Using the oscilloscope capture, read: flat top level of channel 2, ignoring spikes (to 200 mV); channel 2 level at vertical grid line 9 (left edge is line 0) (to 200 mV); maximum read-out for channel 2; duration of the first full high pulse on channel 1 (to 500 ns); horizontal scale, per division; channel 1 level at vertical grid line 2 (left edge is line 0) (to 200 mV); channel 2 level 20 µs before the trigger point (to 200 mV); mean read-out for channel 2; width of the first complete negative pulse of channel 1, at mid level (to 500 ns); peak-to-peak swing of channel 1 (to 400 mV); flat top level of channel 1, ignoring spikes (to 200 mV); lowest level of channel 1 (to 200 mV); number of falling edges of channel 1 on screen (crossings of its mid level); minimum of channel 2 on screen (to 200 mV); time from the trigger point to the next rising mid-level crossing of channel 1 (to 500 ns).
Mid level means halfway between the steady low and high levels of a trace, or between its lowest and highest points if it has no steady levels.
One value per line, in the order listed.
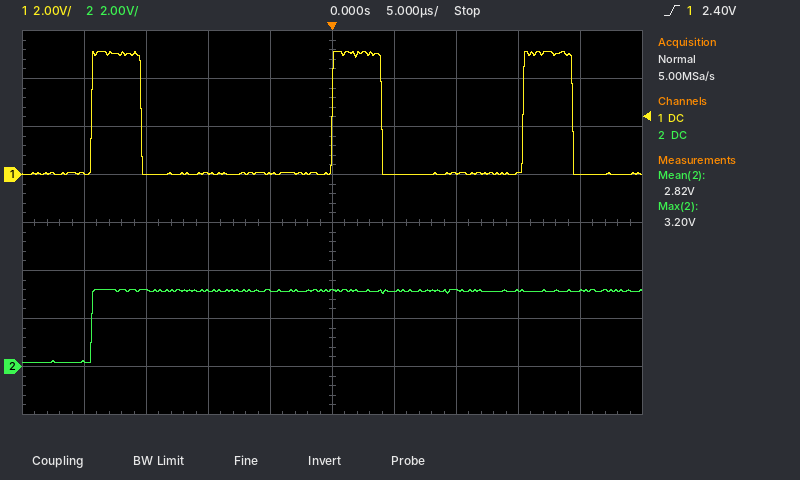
3.2 V
3.2 V
3.20 V
4.0 µs
5 µs
0.0 V
200 mV
2.82 V
15.5 µs
5.2 V
5.0 V
0.0 V
3
200 mV
15.5 µs
